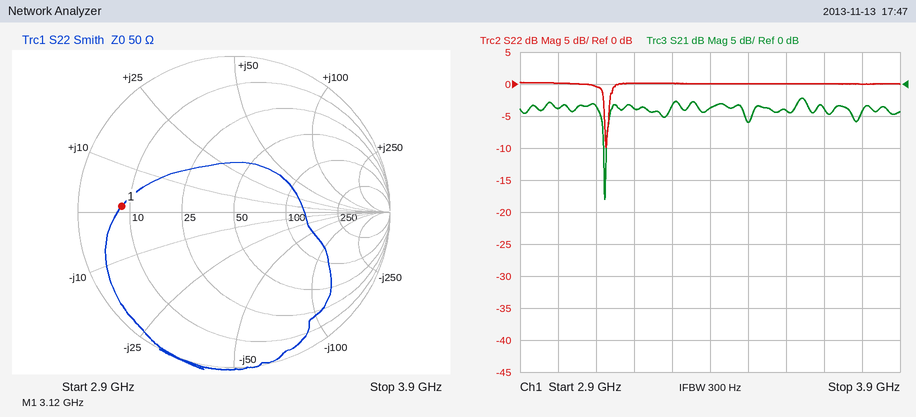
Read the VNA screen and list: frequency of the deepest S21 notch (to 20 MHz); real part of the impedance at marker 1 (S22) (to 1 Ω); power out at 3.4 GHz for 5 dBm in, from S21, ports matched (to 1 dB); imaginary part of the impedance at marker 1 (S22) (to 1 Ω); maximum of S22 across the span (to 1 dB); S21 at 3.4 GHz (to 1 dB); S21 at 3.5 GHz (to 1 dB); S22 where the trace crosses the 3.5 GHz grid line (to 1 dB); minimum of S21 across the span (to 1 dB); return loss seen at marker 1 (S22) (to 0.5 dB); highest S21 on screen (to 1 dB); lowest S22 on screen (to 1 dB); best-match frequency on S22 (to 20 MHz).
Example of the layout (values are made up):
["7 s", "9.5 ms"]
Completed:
["3.12 GHz", "8 Ω", "1 dBm", "+1 Ω", "0 dB", "-4 dB", "-6 dB", "0 dB", "-18 dB", "3.0 dB", "-2 dB", "-10 dB", "3.12 GHz"]
